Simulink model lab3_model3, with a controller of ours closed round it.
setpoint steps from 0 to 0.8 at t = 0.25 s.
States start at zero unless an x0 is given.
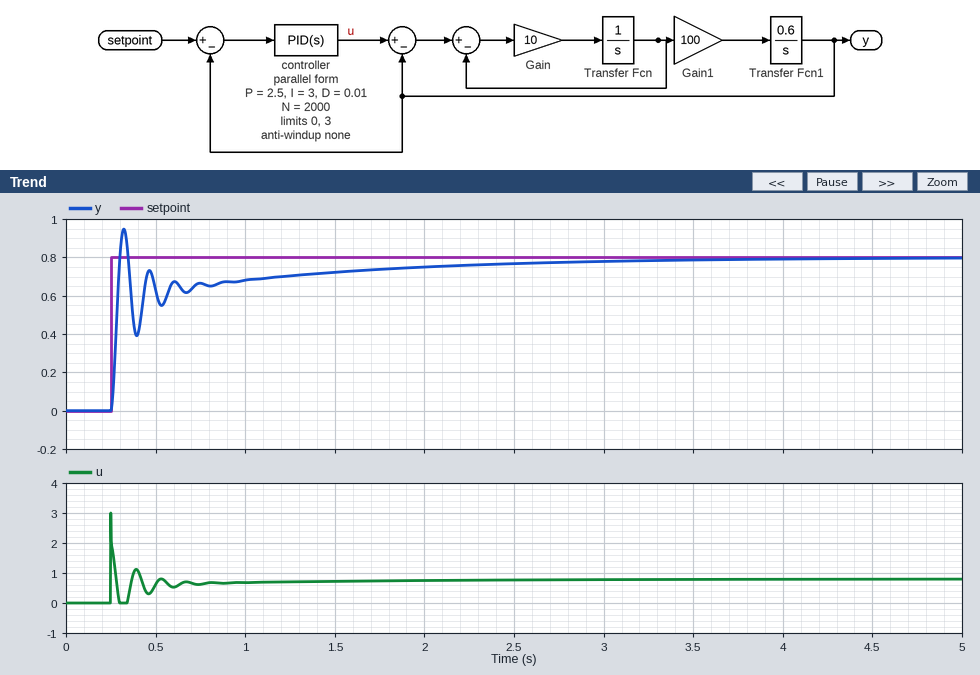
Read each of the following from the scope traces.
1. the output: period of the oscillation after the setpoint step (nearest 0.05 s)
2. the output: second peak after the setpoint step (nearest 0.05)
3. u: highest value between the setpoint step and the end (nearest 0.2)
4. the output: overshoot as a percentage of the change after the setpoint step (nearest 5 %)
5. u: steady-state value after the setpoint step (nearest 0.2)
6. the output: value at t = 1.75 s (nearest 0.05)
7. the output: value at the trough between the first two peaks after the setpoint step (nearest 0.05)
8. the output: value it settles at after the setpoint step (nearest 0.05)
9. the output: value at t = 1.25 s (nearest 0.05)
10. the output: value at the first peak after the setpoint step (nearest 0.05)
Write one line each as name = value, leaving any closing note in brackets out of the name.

the output: period of the oscillation after the setpoint step = 0.15 s
the output: second peak after the setpoint step = 0.75
u: highest value between the setpoint step and the end = 3.0
the output: overshoot as a percentage of the change after the setpoint step = 20 %
u: steady-state value after the setpoint step = 0.8
the output: value at t = 1.75 s = 0.75
the output: value at the trough between the first two peaks after the setpoint step = 0.40
the output: value it settles at after the setpoint step = 0.80
the output: value at t = 1.25 s = 0.70
the output: value at the first peak after the setpoint step = 0.95
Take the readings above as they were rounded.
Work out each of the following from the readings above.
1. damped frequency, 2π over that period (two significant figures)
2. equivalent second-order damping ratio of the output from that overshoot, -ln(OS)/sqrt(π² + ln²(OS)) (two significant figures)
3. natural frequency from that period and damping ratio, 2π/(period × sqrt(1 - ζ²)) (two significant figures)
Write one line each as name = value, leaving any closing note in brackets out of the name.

damped frequency, 2π over that period = 42 rad/s
equivalent second-order damping ratio of the output from that overshoot, -ln(OS)/sqrt(π² + ln²(OS)) = 0.46
natural frequency from that period and damping ratio, 2π/(period × sqrt(1 - ζ²)) = 47 rad/s
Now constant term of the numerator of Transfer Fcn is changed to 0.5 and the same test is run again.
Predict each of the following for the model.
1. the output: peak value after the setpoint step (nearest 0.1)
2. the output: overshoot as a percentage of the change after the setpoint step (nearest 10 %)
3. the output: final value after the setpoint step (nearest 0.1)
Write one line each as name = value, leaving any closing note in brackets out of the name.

the output: peak value after the setpoint step = 1.0
the output: overshoot as a percentage of the change after the setpoint step = 30 %
the output: final value after the setpoint step = 0.8
